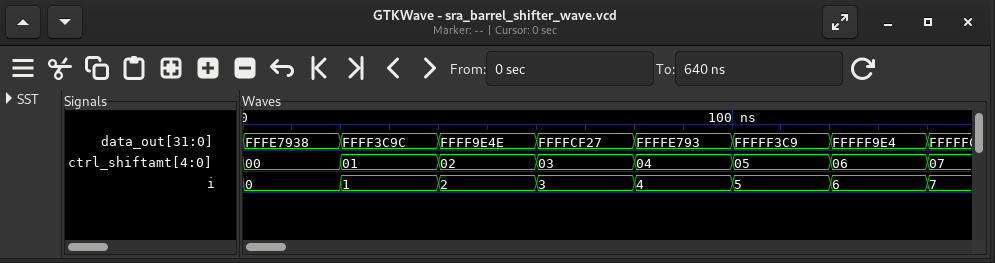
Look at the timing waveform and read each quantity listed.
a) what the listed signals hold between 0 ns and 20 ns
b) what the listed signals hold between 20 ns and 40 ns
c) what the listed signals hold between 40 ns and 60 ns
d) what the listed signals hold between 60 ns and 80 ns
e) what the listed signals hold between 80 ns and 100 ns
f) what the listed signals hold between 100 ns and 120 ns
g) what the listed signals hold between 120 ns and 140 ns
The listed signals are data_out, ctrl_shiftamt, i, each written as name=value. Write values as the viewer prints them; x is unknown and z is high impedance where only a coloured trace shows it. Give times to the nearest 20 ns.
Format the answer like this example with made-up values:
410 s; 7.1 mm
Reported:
data_out=FFFE7938, ctrl_shiftamt=00, i=0; data_out=FFFF3C9C, ctrl_shiftamt=01, i=1; data_out=FFFF9E4E, ctrl_shiftamt=02, i=2; data_out=FFFFCF27, ctrl_shiftamt=03, i=3; data_out=FFFFE793, ctrl_shiftamt=04, i=4; data_out=FFFFF3C9, ctrl_shiftamt=05, i=5; data_out=FFFFF9E4, ctrl_shiftamt=06, i=6
